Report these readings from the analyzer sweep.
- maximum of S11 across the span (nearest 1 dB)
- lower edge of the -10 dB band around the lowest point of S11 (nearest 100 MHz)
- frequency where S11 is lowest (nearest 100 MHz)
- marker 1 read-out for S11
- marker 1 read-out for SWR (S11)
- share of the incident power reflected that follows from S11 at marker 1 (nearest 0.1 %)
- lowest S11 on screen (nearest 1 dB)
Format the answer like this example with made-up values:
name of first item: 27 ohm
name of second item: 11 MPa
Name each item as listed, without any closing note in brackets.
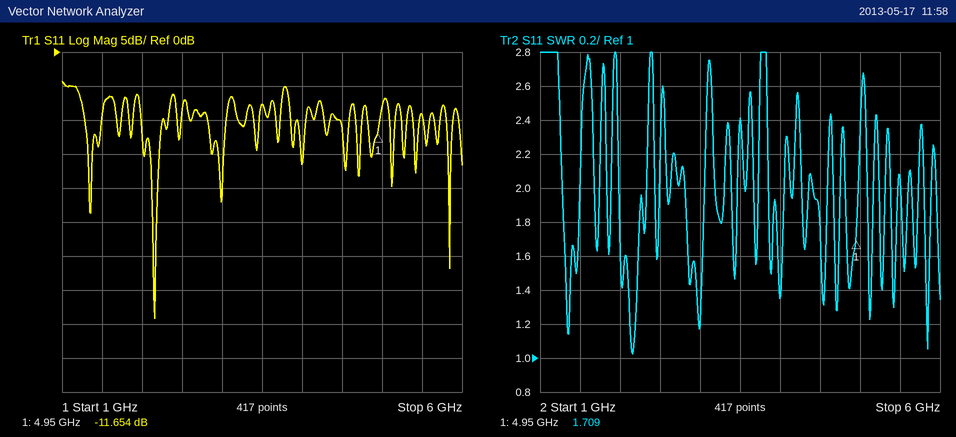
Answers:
maximum of S11 across the span: -4 dB
lower edge of the -10 dB band around the lowest point of S11: 2.0 GHz
frequency where S11 is lowest: 2.2 GHz
marker 1 read-out for S11: -11.654 dB
marker 1 read-out for SWR: 1.709
share of the incident power reflected that follows from S11 at marker 1: 6.8 %
lowest S11 on screen: -39 dB
